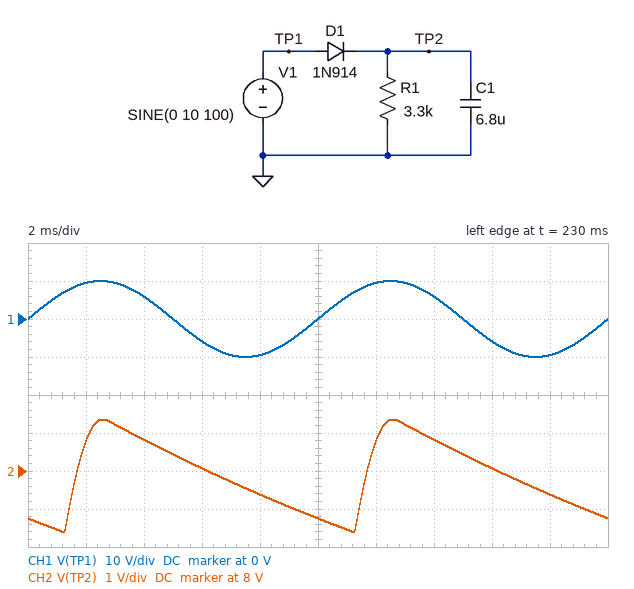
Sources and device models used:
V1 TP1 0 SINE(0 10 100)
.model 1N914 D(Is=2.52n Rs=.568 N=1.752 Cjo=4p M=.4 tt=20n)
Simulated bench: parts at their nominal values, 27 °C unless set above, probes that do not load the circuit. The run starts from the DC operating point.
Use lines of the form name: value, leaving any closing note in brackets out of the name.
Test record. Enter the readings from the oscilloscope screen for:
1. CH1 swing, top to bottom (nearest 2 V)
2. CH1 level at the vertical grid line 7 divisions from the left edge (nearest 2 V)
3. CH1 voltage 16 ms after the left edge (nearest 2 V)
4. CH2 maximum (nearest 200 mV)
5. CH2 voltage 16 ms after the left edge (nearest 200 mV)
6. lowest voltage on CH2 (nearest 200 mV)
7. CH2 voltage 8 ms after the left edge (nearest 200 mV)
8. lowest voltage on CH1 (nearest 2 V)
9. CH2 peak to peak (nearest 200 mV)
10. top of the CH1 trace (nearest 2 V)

CH1 swing, top to bottom: 20 V
CH1 level at the vertical grid line 7 divisions from the left edge: 6 V
CH1 voltage 16 ms after the left edge: -6 V
CH2 maximum: 9.4 V
CH2 voltage 16 ms after the left edge: 8.0 V
lowest voltage on CH2: 6.4 V
CH2 voltage 8 ms after the left edge: 7.4 V
lowest voltage on CH1: -10 V
CH2 peak to peak: 3.0 V
top of the CH1 trace: 10 V
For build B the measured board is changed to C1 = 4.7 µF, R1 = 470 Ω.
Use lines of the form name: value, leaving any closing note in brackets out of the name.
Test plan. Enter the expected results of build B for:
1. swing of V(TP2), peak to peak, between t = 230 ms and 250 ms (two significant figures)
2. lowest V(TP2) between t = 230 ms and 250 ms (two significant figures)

swing of V(TP2), peak to peak, between t = 230 ms and 250 ms: 8.9 V
lowest V(TP2) between t = 230 ms and 250 ms: 370 mV
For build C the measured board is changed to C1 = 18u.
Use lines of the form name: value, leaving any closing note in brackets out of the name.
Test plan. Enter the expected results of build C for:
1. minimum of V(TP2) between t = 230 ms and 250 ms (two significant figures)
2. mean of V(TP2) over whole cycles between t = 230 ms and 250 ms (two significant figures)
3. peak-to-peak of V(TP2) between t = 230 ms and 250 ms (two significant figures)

minimum of V(TP2) between t = 230 ms and 250 ms: 8.0 V
mean of V(TP2) over whole cycles between t = 230 ms and 250 ms: 8.7 V
peak-to-peak of V(TP2) between t = 230 ms and 250 ms: 1.3 V
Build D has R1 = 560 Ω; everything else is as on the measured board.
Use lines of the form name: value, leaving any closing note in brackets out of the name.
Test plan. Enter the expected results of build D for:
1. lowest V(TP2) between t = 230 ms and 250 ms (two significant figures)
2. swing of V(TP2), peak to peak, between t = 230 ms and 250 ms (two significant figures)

lowest V(TP2) between t = 230 ms and 250 ms: 1.3 V
swing of V(TP2), peak to peak, between t = 230 ms and 250 ms: 8.0 V
